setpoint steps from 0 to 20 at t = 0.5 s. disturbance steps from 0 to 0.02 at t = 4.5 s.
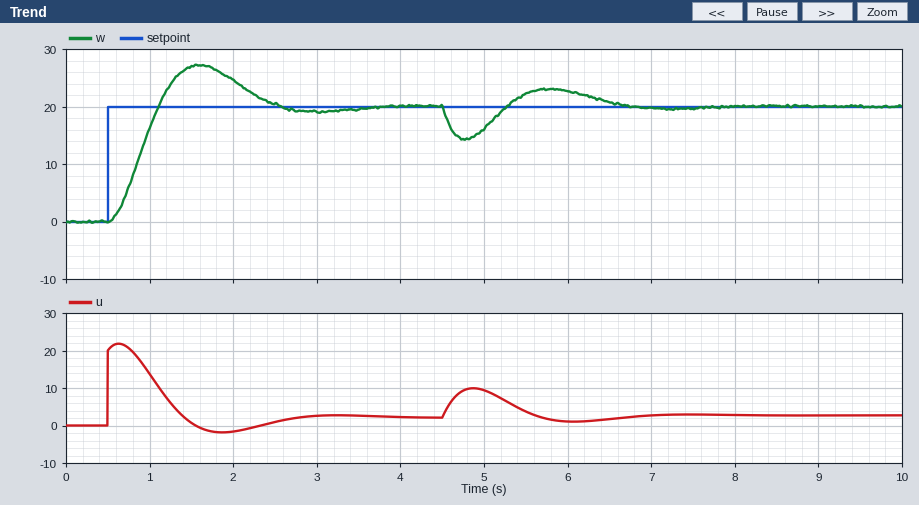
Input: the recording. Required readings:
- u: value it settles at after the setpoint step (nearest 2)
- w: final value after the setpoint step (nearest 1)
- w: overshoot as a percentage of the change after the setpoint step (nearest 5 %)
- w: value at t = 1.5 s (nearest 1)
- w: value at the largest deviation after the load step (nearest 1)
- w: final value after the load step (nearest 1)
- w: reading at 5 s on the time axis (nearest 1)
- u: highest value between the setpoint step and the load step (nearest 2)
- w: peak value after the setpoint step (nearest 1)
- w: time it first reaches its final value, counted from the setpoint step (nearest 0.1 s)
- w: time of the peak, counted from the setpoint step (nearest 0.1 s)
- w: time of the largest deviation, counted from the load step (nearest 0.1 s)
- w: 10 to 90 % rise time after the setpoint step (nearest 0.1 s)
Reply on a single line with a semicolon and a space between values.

2; 20; 35 %; 27; 14; 20; 16; 22; 27; 0.6 s; 1.1 s; 0.3 s; 0.4 s
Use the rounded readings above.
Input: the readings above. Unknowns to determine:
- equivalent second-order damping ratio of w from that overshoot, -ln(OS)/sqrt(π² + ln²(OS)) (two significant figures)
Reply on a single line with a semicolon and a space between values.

0.32
